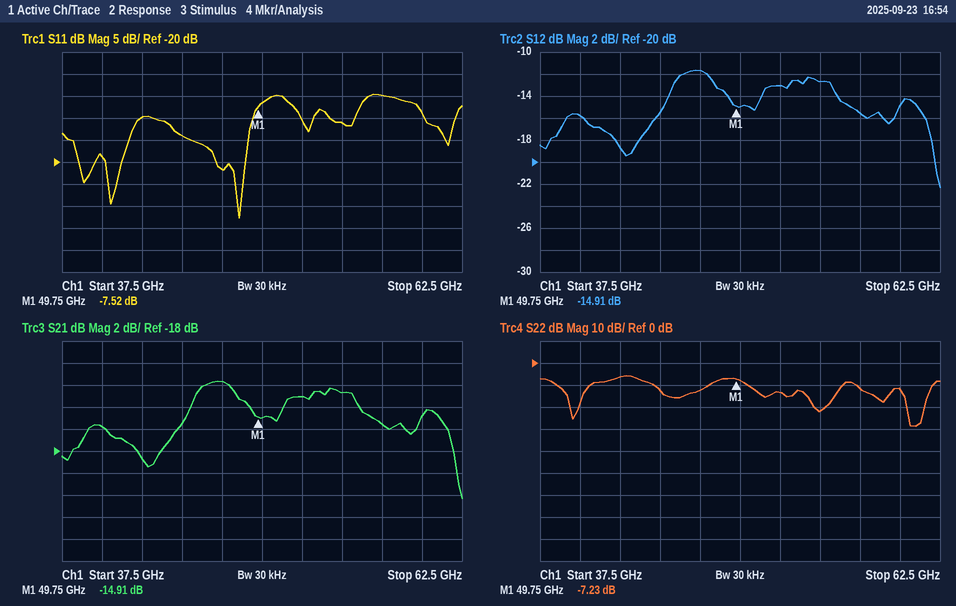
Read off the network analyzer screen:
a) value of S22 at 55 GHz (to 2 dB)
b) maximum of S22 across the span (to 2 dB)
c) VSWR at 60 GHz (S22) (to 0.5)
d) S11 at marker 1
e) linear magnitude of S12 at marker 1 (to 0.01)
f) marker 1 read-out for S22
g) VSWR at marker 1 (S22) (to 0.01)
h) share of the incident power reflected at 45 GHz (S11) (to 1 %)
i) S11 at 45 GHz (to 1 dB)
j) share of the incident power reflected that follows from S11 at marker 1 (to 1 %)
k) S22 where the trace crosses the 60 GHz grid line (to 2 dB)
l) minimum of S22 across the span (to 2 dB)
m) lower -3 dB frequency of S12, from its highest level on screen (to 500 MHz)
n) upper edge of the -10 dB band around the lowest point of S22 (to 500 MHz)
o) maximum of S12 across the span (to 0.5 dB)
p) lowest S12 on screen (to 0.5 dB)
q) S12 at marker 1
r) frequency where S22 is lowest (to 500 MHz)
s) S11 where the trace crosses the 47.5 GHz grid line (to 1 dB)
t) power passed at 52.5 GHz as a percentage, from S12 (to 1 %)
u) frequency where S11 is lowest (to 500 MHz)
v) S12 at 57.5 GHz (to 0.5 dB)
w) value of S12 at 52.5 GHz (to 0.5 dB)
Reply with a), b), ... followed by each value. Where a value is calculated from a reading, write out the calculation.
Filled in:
a) -22 dB
b) -6 dB
c) |Γ| = 10^(-12/20) = 0.2512; VSWR = (1 + 0.2512)/(1 − 0.2512) ≈ 1.67, so 1.5 to the nearest 0.5
d) -7.52 dB
e) 10^(-14.91/20) ≈ 0.18
f) -7.23 dB
g) (1 + 0.4350)/(1 − 0.4350) ≈ 2.54
h) 10^(-14/10) ≈ 4 %
i) -14 dB
j) 10^(-7.52/10) ≈ 18 %
k) -12 dB
l) -28 dB
m) 45.5 GHz
n) 62.0 GHz
o) -11.5 dB
p) -22.5 dB
q) -14.91 dB
r) 61.0 GHz
s) -22 dB
t) 10^(-13/10) ≈ 5 %
u) 48.5 GHz
v) -15.5 dB
w) -13.0 dB
